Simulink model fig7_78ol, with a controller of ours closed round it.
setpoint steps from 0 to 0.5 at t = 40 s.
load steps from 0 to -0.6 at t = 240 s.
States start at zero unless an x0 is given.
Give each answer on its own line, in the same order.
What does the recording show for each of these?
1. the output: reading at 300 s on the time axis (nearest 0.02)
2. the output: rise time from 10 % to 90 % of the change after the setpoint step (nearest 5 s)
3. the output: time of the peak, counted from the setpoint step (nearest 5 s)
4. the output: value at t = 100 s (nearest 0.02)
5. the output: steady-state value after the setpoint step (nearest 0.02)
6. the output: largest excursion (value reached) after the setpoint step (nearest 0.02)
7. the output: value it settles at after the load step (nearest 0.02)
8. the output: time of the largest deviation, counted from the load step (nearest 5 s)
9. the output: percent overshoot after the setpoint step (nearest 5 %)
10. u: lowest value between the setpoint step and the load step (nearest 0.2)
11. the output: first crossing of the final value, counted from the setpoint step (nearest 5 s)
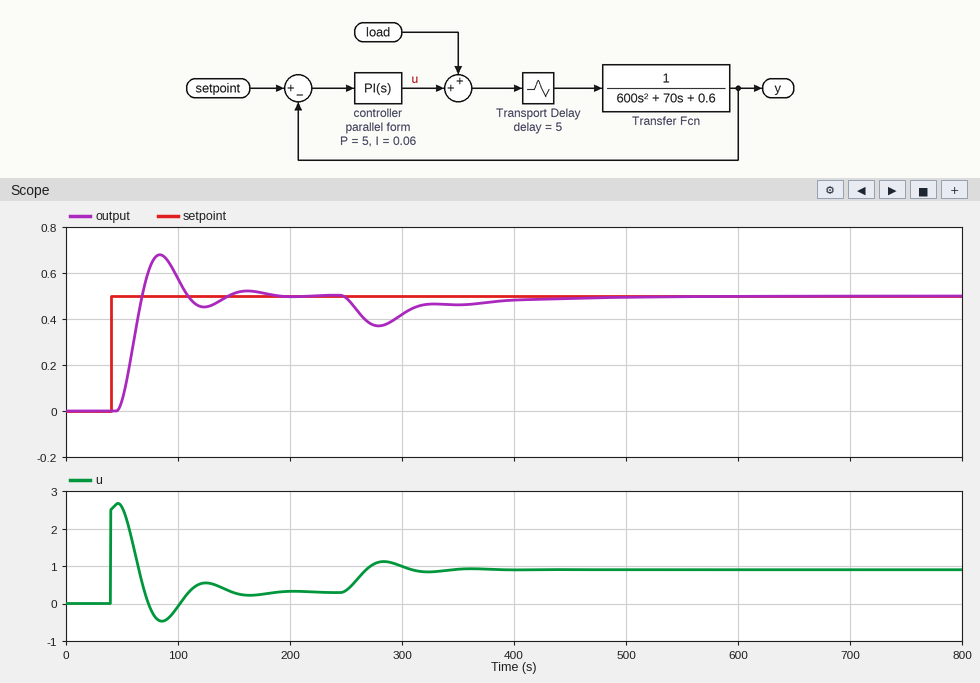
0.42
15 s
45 s
0.58
0.50
0.68
0.50
40 s
35 %
-0.4
30 s
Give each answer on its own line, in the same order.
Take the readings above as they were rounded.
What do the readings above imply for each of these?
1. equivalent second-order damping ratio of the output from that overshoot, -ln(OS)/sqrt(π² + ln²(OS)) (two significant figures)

0.32
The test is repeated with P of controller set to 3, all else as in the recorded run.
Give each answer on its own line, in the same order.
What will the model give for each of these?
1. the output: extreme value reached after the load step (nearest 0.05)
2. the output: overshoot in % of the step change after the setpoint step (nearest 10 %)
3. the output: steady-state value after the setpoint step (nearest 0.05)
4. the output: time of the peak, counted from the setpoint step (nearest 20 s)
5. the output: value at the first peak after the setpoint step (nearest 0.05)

0.35
30 %
0.50
60 s
0.65
